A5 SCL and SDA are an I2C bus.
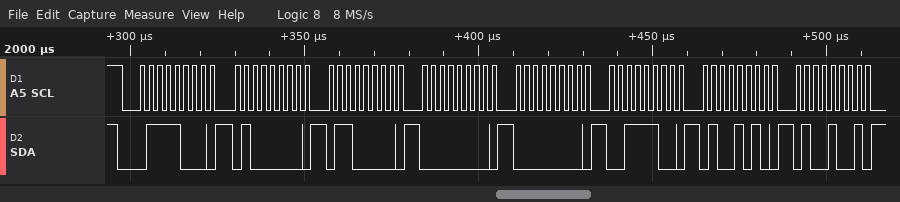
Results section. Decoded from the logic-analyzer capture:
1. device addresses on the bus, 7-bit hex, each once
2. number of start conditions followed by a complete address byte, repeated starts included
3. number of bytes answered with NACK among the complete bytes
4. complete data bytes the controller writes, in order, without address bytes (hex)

0x3C
1
0
40 60 00 00 3C 4A 49
